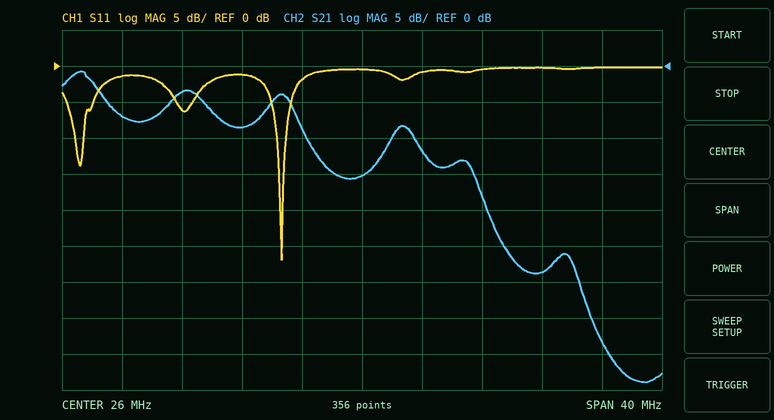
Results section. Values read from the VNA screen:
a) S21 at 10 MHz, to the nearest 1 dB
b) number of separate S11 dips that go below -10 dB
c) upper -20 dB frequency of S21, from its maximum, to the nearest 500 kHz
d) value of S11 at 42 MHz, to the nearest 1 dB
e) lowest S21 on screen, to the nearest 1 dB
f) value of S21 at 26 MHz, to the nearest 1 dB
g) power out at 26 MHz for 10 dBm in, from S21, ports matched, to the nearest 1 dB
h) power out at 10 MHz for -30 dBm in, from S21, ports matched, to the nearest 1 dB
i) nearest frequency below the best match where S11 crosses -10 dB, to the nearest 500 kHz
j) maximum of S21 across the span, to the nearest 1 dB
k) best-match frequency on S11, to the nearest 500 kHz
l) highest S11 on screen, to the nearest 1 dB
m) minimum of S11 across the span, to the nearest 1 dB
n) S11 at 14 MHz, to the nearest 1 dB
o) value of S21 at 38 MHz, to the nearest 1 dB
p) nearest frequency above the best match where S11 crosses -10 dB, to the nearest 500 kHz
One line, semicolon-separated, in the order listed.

-7 dB; 2; 34.5 MHz; 0 dB; -44 dB; -15 dB; -5 dBm; -37 dBm; 20.5 MHz; -1 dB; 20.5 MHz; 0 dB; -27 dB; -6 dB; -29 dB; 21.0 MHz
